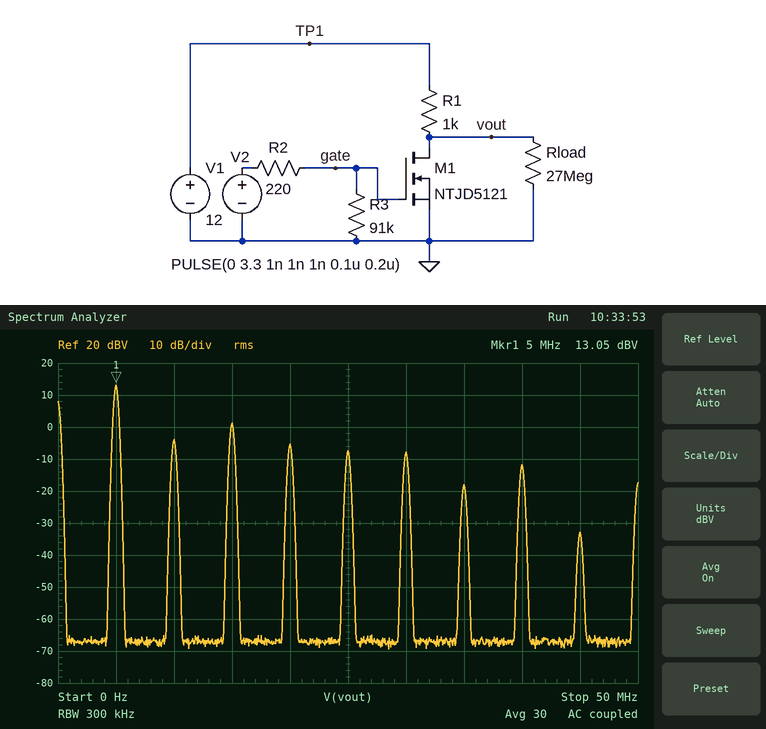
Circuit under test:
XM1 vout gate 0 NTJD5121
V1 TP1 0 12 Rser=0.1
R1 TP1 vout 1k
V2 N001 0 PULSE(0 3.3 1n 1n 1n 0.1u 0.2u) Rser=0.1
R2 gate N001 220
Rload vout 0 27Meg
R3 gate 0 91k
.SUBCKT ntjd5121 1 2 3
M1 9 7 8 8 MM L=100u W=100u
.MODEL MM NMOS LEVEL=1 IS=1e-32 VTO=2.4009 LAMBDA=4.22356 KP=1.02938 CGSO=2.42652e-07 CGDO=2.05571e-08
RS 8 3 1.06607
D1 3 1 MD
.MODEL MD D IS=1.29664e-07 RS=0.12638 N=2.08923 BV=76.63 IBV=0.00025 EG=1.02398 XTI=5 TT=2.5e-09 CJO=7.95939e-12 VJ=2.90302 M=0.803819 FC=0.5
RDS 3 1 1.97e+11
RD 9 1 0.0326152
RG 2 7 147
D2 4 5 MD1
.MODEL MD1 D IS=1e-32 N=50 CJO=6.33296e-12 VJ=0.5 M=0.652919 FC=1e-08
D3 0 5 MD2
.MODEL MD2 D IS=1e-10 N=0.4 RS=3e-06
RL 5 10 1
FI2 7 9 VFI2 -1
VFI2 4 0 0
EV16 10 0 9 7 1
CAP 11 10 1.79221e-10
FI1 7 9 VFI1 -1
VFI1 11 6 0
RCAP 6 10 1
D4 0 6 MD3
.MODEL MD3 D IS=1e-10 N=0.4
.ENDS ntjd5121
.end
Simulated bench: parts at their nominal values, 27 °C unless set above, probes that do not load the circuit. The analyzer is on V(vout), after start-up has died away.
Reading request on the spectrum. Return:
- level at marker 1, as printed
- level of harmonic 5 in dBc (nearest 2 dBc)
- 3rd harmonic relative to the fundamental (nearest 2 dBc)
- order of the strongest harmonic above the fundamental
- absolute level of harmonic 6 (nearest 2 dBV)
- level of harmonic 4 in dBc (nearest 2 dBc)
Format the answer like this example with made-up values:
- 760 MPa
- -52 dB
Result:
- 13.05 dBV
- -20 dBc
- -12 dBc
- 3
- -8 dBV
- -18 dBc
